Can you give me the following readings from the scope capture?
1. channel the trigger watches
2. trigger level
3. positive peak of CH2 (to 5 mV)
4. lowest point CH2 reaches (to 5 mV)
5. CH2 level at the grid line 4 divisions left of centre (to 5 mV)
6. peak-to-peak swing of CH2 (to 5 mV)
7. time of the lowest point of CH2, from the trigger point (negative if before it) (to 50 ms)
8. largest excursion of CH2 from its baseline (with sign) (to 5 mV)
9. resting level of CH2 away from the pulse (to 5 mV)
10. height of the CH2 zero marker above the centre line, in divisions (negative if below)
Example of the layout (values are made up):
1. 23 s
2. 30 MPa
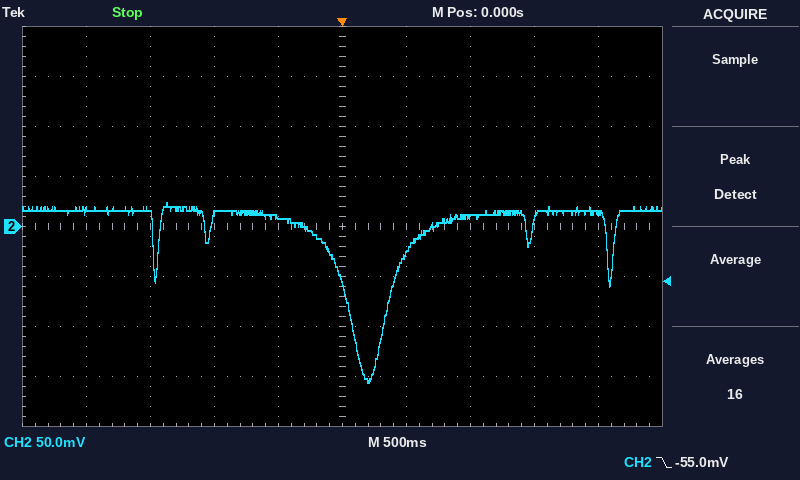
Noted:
1. CH2
2. -55.0 mV
3. 25 mV
4. -155 mV
5. 15 mV
6. 180 mV
7. +200 ms
8. -170 mV
9. 15 mV
10. 0.0 div
